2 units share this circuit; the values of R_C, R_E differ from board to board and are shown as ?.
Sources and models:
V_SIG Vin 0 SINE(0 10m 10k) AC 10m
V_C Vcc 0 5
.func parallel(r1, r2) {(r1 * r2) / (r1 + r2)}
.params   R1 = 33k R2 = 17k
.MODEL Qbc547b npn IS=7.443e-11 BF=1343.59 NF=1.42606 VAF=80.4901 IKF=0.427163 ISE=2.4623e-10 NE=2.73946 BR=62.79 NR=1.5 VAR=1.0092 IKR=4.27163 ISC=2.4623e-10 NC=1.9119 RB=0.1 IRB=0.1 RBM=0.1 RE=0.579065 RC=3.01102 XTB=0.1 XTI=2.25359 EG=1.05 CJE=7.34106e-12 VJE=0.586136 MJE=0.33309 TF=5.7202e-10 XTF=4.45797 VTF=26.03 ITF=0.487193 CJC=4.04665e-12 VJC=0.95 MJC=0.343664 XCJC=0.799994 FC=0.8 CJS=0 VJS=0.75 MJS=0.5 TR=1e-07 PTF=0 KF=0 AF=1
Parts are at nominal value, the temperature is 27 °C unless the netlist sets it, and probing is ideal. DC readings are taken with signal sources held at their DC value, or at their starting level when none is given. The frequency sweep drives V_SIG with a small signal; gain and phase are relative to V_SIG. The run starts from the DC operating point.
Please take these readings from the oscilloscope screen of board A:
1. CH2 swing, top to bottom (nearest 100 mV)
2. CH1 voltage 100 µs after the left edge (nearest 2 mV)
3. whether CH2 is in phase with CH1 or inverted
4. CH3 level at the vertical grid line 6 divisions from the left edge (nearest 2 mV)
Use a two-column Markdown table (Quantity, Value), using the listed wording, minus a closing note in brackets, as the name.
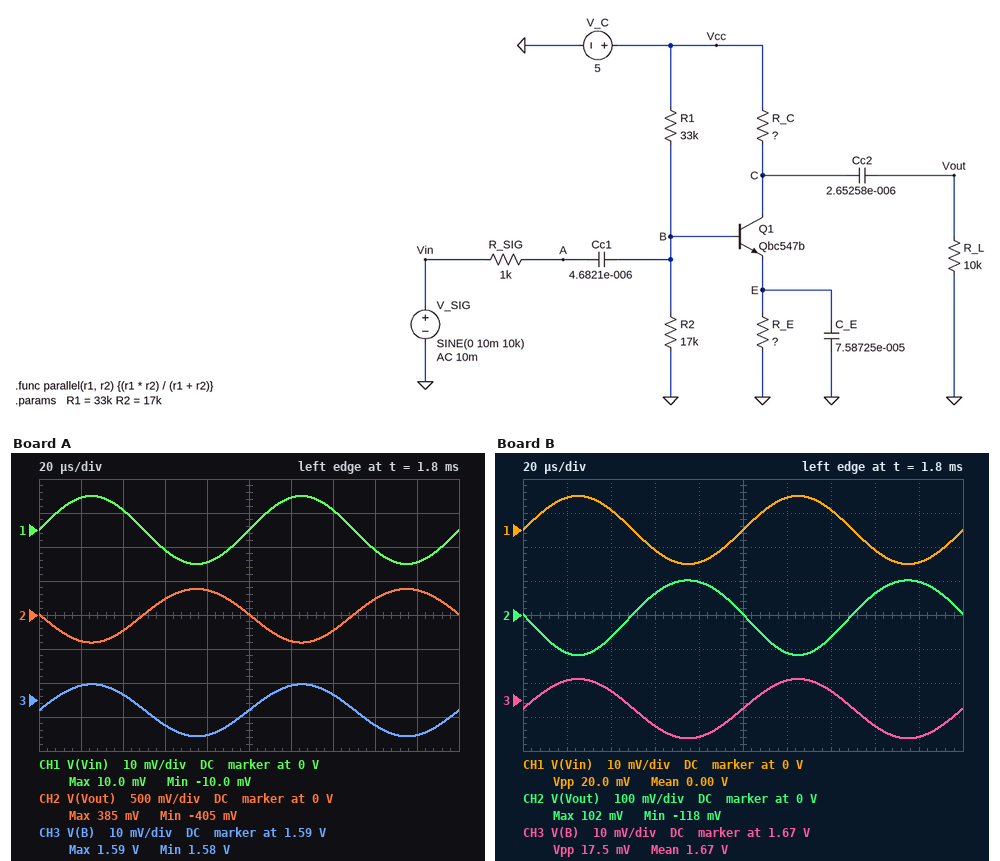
| Quantity | Value |
|---|---|
| CH2 swing, top to bottom | 800 mV |
| CH1 voltage 100 µs after the left edge | 0 V |
| whether CH2 is in phase with CH1 or inverted | inverted |
| CH3 level at the vertical grid line 6 divisions from the left edge | 1.594 V |
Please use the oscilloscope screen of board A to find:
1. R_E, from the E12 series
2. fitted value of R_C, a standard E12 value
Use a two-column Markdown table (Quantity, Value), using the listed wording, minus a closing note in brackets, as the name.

| Quantity | Value |
|---|---|
| R_E, from the E12 series | 330 Ω |
| fitted value of R_C, a standard E12 value | 1 kΩ |
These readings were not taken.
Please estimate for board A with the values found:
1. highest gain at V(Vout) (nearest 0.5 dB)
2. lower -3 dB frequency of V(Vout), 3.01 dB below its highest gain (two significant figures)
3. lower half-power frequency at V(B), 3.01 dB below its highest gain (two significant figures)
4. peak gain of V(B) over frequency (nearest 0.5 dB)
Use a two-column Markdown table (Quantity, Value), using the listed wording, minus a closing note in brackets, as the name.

| Quantity | Value |
|---|---|
| highest gain at V(Vout) | 32.0 dB |
| lower -3 dB frequency of V(Vout), 3.01 dB below its highest gain | 110 Hz |
| lower half-power frequency at V(B), 3.01 dB below its highest gain | 2.9 Hz |
| peak gain of V(B) over frequency | -1.5 dB |
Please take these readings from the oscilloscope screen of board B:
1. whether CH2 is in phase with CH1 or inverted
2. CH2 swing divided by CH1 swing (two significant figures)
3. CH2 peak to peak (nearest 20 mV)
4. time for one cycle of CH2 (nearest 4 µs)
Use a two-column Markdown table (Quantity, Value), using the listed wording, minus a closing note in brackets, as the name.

| Quantity | Value |
|---|---|
| whether CH2 is in phase with CH1 or inverted | inverted |
| CH2 swing divided by CH1 swing | 11 |
| CH2 peak to peak | 220 mV |
| time for one cycle of CH2 | 100 µs |
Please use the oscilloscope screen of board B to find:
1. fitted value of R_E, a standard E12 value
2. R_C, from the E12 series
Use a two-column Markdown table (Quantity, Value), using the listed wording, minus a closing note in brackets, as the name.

| Quantity | Value |
|---|---|
| fitted value of R_E, a standard E12 value | 1.5 kΩ |
| R_C, from the E12 series | 820 Ω |
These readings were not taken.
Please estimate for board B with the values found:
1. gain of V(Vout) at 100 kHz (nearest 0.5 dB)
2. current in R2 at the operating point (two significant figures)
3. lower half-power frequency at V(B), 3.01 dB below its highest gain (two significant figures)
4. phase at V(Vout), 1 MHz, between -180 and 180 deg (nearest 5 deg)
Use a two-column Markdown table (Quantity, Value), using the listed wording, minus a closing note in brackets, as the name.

| Quantity | Value |
|---|---|
| gain of V(Vout) at 100 kHz | 21.0 dB |
| current in R2 at the operating point | 98 µA |
| lower half-power frequency at V(B), 3.01 dB below its highest gain | 2.7 Hz |
| phase at V(Vout), 1 MHz, between -180 and 180 deg | 160 deg |
